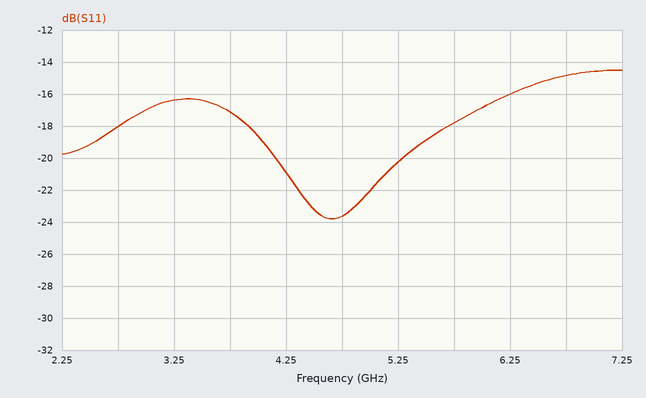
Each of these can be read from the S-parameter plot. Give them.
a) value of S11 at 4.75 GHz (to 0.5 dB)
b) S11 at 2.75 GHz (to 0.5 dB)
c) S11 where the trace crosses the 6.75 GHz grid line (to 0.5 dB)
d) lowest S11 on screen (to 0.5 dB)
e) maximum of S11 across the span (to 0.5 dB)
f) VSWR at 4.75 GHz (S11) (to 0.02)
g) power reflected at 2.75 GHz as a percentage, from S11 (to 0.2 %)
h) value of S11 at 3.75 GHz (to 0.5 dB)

-23.5 dB
-18.0 dB
-15.0 dB
-24.0 dB
-14.5 dB
1.14
1.6 %
-17.0 dB
